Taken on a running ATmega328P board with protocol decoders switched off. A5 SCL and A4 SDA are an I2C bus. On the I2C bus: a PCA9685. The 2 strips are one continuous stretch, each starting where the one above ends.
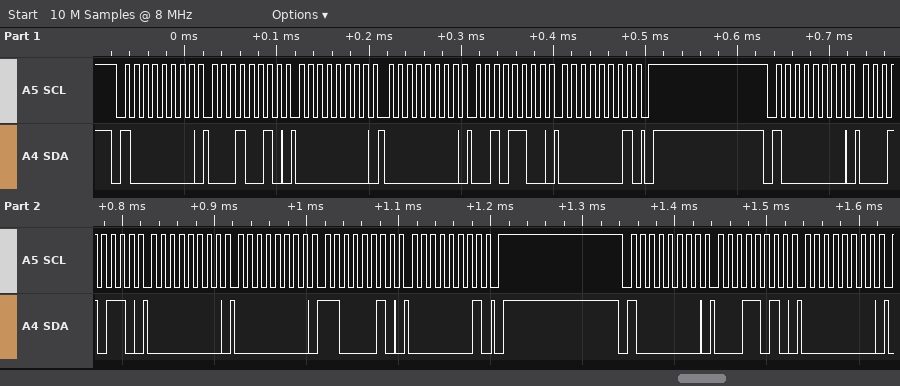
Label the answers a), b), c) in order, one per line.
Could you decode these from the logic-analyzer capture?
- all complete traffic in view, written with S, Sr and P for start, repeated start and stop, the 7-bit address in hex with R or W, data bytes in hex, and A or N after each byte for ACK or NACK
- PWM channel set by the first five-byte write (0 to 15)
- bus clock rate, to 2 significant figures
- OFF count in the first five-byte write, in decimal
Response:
a) S 40W A 12 A 00 A 00 A 2C A 01 A P S 40W A 16 A 00 A 00 A C2 A 01 A P S 40W A 1A A 00 A
b) 3
c) 100 kHz
d) 300
